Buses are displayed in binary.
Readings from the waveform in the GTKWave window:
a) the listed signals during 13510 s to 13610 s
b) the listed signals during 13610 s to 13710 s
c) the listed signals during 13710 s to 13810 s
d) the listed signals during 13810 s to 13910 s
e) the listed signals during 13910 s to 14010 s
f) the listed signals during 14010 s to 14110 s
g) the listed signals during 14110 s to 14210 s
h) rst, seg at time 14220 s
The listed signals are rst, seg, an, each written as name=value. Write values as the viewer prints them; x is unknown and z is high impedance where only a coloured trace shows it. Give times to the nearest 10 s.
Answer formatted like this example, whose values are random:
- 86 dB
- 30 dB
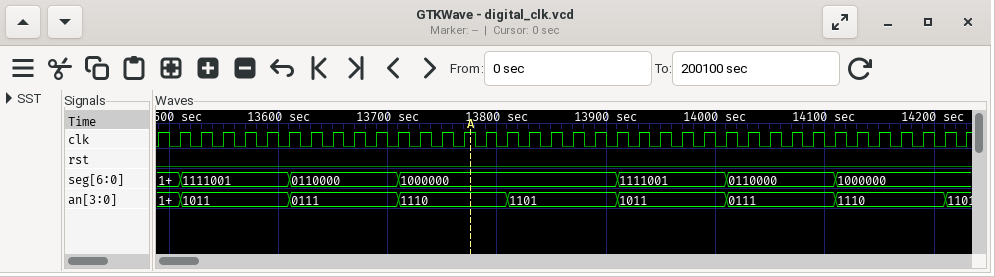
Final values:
- rst=0, seg=1111001, an=1011
- rst=0, seg=0110000, an=0111
- rst=0, seg=1000000, an=1110
- rst=0, seg=1000000, an=1101
- rst=0, seg=1111001, an=1011
- rst=0, seg=0110000, an=0111
- rst=0, seg=1000000, an=1110
- rst=0, seg=1000000
